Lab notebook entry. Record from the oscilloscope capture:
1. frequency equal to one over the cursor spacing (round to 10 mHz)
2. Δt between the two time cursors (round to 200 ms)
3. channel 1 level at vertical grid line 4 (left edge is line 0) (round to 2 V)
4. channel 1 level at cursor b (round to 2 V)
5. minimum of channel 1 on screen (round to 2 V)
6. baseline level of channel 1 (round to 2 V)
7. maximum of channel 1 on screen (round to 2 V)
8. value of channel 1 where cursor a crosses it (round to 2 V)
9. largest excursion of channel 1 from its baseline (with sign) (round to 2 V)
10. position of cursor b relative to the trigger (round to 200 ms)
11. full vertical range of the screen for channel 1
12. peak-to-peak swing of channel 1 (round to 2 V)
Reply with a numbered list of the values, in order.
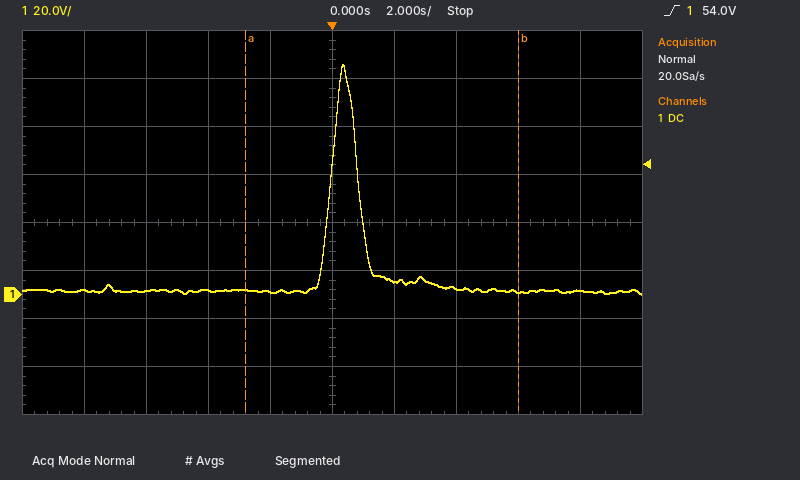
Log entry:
1. 110 mHz
2. 8.8 s
3. 2 V
4. 2 V
5. 0 V
6. 2 V
7. 96 V
8. 2 V
9. +94 V
10. +6.0 s
11. 160 V
12. 96 V
